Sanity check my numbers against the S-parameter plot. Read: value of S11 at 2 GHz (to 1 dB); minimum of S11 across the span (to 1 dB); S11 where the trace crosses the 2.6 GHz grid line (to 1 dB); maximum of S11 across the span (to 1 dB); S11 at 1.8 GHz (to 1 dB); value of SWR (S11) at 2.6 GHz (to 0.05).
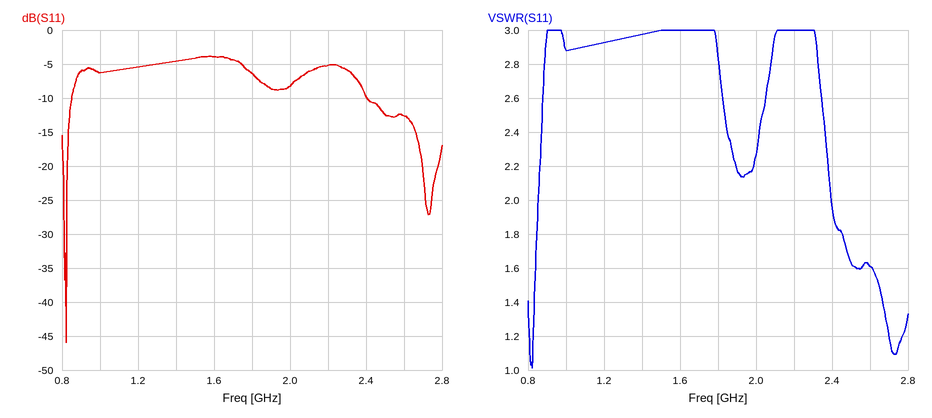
-8 dB
-46 dB
-13 dB
-4 dB
-6 dB
1.60
